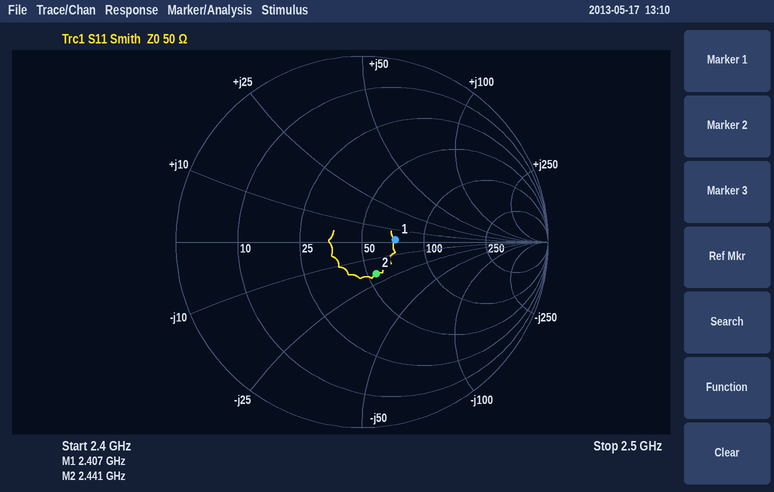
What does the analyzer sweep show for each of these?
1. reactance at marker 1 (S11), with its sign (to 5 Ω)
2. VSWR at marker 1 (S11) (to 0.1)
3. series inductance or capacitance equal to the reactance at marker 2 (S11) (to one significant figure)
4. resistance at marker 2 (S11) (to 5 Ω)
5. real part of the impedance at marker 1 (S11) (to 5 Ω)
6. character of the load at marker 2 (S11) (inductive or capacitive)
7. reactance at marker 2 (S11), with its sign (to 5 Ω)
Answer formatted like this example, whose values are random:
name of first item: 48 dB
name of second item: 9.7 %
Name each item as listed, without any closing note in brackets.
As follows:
reactance at marker 1 (S11), with its sign: 0 Ω
VSWR at marker 1 (S11): 1.4
series inductance or capacitance equal to the reactance at marker 2 (S11): 3 pF
resistance at marker 2 (S11): 55 Ω
real part of the impedance at marker 1 (S11): 70 Ω
character of the load at marker 2 (S11): capacitive
reactance at marker 2 (S11), with its sign: -20 Ω
